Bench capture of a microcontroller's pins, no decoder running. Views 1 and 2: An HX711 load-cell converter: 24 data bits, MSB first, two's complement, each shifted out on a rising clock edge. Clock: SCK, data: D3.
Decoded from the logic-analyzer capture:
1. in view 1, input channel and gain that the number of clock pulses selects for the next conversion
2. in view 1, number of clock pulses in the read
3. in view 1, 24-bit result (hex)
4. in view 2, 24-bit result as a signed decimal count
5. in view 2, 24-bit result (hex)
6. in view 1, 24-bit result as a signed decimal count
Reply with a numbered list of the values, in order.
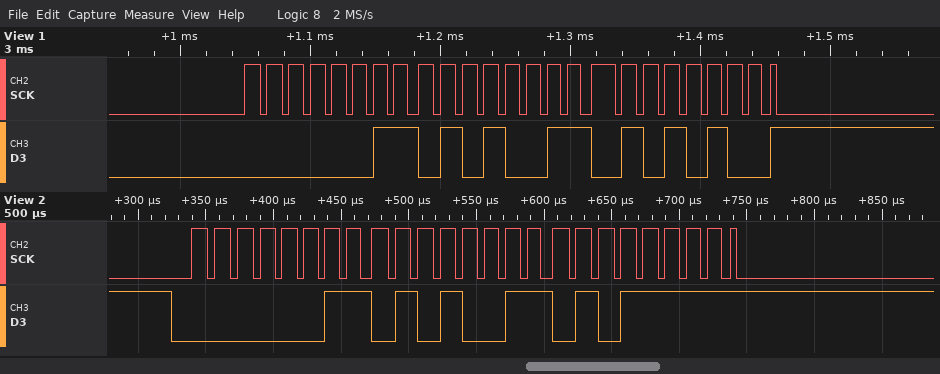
1. channel A, gain 128
2. 25
3. 0x035354
4. 217951
5. 0x03535F
6. 217940
